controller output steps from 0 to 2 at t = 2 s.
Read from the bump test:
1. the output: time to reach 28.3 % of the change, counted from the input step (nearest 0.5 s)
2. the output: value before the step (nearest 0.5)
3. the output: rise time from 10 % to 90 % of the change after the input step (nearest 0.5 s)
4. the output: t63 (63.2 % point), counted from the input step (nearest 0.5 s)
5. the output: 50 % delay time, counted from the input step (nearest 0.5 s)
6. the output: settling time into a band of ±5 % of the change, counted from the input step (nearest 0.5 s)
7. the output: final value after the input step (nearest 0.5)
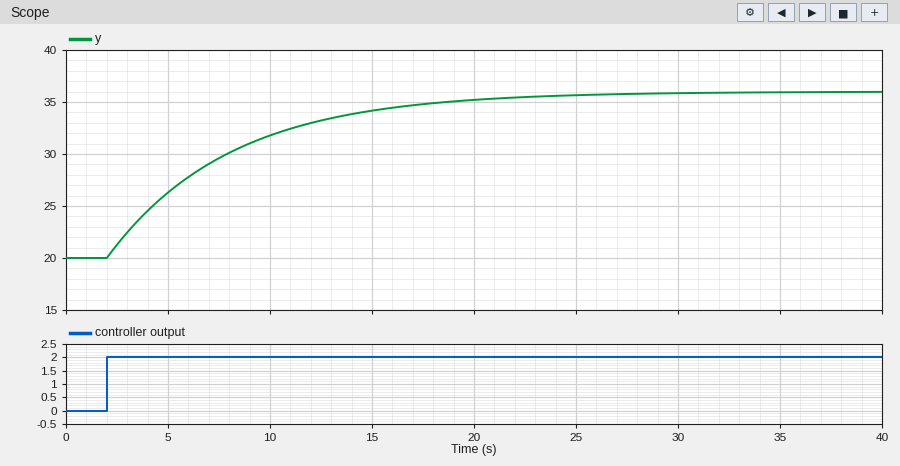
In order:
2.0 s
20.0
13.0 s
6.0 s
4.0 s
18.0 s
36.0
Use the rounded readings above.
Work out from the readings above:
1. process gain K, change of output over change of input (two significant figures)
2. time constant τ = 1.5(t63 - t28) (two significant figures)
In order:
8.0
6.0 s
